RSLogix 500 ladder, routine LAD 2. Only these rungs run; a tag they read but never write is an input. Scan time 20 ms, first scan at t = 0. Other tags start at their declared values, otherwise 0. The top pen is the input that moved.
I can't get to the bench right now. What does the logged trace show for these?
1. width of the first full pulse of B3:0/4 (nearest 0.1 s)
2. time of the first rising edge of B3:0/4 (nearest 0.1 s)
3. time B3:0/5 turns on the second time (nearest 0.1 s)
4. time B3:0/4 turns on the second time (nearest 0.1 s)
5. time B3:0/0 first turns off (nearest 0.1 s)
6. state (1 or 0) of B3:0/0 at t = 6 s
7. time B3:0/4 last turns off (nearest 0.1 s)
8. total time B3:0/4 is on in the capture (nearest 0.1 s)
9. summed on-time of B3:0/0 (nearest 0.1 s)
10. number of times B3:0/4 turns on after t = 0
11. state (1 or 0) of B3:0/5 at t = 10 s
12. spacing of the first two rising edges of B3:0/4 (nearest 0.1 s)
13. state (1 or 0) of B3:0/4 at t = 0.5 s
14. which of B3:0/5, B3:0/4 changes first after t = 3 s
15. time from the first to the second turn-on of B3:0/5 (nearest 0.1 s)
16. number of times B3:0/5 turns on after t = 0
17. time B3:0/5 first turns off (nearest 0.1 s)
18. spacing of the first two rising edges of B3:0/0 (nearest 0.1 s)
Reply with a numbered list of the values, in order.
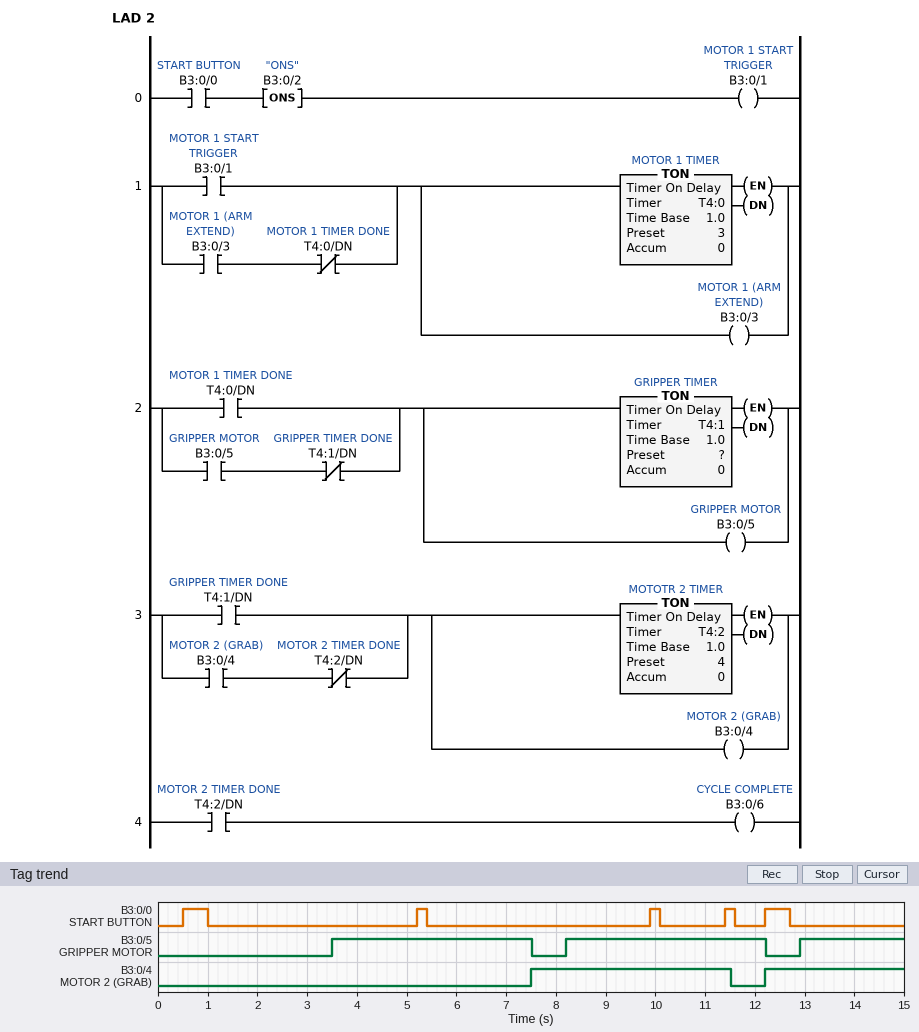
1. 4.0 s
2. 7.5 s
3. 8.2 s
4. 12.2 s
5. 1.0 s
6. 0
7. 11.5 s
8. 6.8 s
9. 1.6 s
10. 2
11. 1
12. 4.7 s
13. 0
14. B3:0/5
15. 4.7 s
16. 3
17. 7.5 s
18. 4.7 s
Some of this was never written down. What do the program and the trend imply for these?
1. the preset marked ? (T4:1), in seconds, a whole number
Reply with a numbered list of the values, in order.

1. 4 s
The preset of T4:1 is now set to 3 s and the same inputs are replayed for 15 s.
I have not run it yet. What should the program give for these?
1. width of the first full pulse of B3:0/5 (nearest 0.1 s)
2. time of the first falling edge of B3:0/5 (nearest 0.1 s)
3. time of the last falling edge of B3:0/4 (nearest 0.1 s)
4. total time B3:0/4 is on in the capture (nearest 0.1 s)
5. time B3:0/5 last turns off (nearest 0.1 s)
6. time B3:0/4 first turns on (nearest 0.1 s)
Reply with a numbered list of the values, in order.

1. 3.0 s
2. 6.5 s
3. 10.5 s
4. 7.8 s
5. 11.2 s
6. 6.5 s
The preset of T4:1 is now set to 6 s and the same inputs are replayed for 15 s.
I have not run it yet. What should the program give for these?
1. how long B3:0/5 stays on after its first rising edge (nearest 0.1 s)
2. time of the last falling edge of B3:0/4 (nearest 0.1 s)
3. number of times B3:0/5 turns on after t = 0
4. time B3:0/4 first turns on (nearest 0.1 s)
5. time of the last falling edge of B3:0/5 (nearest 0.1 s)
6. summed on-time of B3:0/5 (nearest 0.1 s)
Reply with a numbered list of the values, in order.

1. 6.0 s
2. 13.5 s
3. 2
4. 9.5 s
5. 9.5 s
6. 8.1 s
